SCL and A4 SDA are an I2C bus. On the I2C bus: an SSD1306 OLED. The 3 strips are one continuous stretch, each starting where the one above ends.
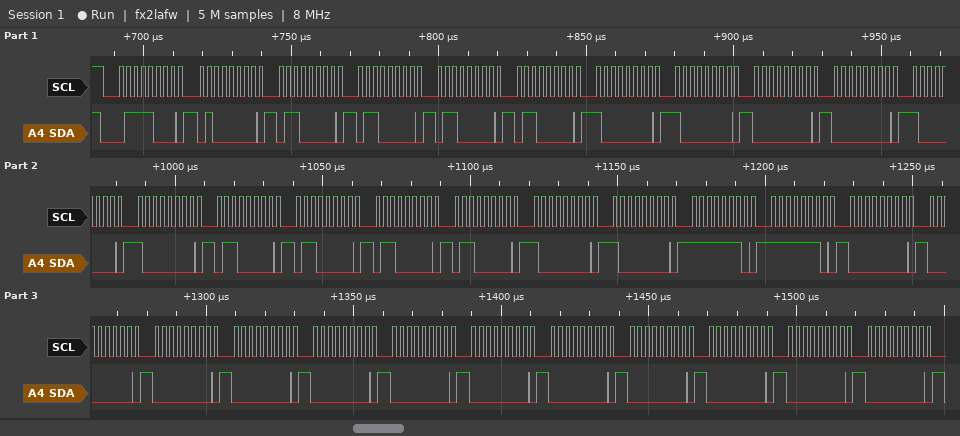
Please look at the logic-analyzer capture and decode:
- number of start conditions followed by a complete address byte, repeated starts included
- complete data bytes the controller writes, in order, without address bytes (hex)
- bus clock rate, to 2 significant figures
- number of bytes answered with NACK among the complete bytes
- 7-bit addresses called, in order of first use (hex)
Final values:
1
40 60 60 60 60 80 80 00 00 80 80 60 60 60 60 80 80 FE FE 00 00 00 00 00 00 00 00 00 00 00 00
400 kHz
0
0x3C
